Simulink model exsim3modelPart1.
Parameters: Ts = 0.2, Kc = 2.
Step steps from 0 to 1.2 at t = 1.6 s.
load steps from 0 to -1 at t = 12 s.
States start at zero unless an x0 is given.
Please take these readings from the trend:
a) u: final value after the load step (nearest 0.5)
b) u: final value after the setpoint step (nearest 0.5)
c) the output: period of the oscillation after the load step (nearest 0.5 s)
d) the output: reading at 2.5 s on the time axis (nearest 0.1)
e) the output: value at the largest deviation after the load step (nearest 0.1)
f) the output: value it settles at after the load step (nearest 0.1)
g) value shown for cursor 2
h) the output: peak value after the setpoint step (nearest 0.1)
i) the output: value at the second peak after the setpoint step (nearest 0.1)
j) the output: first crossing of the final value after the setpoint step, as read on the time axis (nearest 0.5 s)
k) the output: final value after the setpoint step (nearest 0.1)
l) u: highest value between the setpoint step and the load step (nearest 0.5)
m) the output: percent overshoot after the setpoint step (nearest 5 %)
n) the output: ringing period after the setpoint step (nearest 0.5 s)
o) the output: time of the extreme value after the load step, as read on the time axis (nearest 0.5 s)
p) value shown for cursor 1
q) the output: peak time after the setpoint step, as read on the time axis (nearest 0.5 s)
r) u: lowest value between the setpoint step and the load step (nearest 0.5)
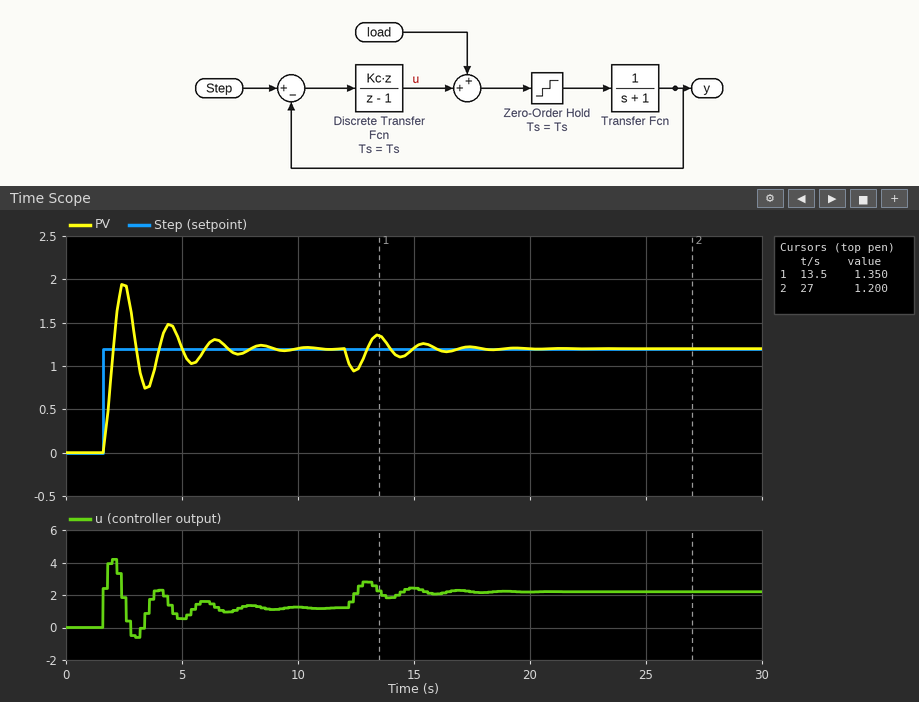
2.0
1.0
2.0 s
1.9
0.9
1.2
1.200
1.9
1.5
2.0 s
1.2
4.0
60 %
2.0 s
12.5 s
1.350
2.5 s
-0.5
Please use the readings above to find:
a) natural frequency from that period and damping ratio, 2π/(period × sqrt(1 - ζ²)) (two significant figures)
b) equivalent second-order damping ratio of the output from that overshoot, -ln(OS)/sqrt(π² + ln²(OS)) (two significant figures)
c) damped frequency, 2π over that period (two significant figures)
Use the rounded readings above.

3.2 rad/s
0.16
3.1 rad/s
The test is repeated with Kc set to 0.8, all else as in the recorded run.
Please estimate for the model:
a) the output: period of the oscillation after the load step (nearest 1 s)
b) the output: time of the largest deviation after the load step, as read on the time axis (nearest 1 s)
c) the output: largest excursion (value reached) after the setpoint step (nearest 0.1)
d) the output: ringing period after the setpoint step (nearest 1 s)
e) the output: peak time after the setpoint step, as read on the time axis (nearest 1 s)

3 s
13 s
1.7
3 s
3 s
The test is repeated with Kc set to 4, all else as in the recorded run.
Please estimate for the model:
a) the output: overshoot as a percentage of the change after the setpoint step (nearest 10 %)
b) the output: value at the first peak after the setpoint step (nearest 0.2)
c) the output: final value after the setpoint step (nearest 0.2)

80 %
2.2
1.2
